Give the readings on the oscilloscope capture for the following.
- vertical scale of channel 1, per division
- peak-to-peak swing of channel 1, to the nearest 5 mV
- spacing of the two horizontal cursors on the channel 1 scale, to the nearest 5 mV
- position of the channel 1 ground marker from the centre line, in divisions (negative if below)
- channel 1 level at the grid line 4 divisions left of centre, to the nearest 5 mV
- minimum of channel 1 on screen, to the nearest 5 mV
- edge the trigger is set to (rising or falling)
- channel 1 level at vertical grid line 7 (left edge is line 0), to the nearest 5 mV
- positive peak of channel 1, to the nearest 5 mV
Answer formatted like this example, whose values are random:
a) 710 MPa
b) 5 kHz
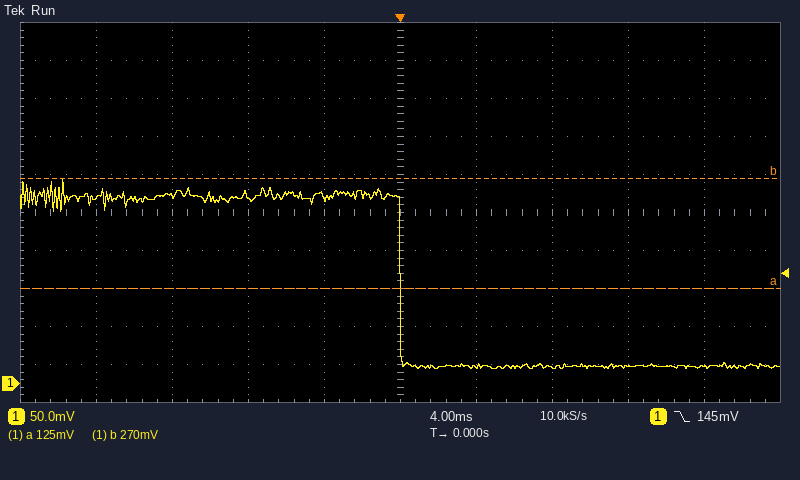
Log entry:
a) 50 mV
b) 250 mV
c) 145 mV
d) -4.5 div
e) 245 mV
f) 20 mV
g) falling
h) 20 mV
i) 270 mV
